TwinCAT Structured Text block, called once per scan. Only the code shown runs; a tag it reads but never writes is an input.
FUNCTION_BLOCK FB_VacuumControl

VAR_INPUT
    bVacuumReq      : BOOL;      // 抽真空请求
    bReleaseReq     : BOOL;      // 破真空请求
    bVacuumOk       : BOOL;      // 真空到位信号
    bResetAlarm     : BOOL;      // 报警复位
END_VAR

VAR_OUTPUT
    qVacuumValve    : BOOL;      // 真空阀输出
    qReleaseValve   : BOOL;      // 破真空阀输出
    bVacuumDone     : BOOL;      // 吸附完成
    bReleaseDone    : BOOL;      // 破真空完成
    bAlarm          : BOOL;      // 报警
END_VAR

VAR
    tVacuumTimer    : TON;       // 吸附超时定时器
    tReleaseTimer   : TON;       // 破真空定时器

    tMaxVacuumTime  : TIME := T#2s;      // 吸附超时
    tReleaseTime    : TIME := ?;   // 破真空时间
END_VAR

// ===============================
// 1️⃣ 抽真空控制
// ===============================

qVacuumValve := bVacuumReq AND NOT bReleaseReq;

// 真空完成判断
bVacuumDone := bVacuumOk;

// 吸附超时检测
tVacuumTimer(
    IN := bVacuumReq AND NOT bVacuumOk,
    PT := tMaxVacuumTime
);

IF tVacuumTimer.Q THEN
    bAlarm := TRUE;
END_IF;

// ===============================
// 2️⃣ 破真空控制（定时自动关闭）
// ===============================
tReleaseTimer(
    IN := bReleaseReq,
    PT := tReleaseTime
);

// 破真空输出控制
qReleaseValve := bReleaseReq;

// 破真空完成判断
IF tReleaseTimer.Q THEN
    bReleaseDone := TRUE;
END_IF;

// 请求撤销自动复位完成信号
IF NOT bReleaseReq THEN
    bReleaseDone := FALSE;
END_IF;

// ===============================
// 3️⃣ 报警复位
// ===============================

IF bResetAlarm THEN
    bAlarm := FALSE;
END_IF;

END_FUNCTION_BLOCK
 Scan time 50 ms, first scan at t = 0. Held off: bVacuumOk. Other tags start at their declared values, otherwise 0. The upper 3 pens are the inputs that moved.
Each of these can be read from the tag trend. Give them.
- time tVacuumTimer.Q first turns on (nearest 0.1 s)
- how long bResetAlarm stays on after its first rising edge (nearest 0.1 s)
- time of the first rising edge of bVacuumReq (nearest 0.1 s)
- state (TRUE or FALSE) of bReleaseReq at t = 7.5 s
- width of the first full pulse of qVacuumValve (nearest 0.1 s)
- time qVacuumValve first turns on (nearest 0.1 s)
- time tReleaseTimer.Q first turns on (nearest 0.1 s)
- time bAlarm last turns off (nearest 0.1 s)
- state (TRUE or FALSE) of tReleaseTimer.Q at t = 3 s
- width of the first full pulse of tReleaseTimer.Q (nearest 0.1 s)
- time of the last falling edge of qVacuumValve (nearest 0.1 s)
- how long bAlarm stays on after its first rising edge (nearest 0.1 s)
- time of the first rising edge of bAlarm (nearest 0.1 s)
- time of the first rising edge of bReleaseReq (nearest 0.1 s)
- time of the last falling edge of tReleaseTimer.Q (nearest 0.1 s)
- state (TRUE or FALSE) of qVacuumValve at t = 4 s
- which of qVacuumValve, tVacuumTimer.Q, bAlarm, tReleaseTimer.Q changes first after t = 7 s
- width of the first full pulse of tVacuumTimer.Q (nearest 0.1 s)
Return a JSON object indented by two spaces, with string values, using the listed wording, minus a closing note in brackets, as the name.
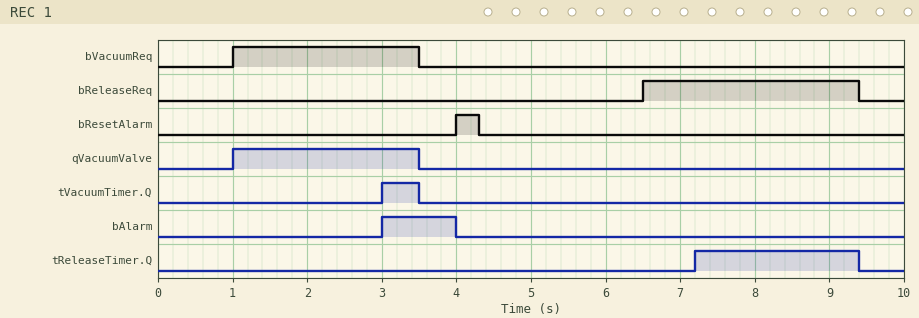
{
  "time tVacuumTimer.Q first turns on": "3.0 s",
  "how long bResetAlarm stays on after its first rising edge": "0.3 s",
  "time of the first rising edge of bVacuumReq": "1.0 s",
  "state (TRUE or FALSE) of bReleaseReq at t = 7.5 s": "TRUE",
  "width of the first full pulse of qVacuumValve": "2.5 s",
  "time qVacuumValve first turns on": "1.0 s",
  "time tReleaseTimer.Q first turns on": "7.2 s",
  "time bAlarm last turns off": "4.0 s",
  "state (TRUE or FALSE) of tReleaseTimer.Q at t = 3 s": "FALSE",
  "width of the first full pulse of tReleaseTimer.Q": "2.2 s",
  "time of the last falling edge of qVacuumValve": "3.5 s",
  "how long bAlarm stays on after its first rising edge": "1.0 s",
  "time of the first rising edge of bAlarm": "3.0 s",
  "time of the first rising edge of bReleaseReq": "6.5 s",
  "time of the last falling edge of tReleaseTimer.Q": "9.4 s",
  "state (TRUE or FALSE) of qVacuumValve at t = 4 s": "FALSE",
  "which of qVacuumValve, tVacuumTimer.Q, bAlarm, tReleaseTimer.Q changes first after t = 7 s": "tReleaseTimer.Q",
  "width of the first full pulse of tVacuumTimer.Q": "0.5 s"
}
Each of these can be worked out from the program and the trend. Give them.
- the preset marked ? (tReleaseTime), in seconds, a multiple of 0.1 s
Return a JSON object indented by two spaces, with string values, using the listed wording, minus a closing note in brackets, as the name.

{
  "the preset marked ? (tReleaseTime), in seconds, a multiple of 0.1 s": "0.7 s"
}
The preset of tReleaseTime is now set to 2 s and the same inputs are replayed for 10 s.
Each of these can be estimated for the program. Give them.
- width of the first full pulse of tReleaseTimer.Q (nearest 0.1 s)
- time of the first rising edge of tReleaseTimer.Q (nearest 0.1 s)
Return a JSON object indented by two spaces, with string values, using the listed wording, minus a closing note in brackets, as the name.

{
  "width of the first full pulse of tReleaseTimer.Q": "0.9 s",
  "time of the first rising edge of tReleaseTimer.Q": "8.5 s"
}
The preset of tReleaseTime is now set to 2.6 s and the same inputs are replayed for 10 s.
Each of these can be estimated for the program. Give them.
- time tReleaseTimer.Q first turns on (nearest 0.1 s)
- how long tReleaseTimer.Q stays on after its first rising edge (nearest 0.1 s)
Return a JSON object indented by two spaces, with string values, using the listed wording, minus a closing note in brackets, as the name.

{
  "time tReleaseTimer.Q first turns on": "9.1 s",
  "how long tReleaseTimer.Q stays on after its first rising edge": "0.3 s"
}
